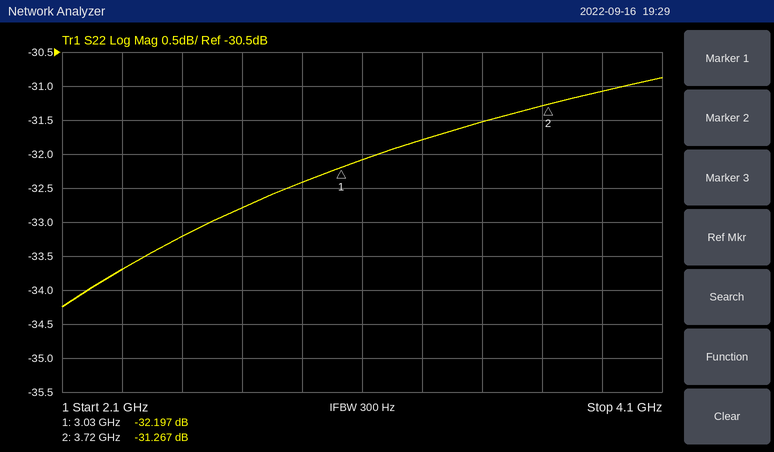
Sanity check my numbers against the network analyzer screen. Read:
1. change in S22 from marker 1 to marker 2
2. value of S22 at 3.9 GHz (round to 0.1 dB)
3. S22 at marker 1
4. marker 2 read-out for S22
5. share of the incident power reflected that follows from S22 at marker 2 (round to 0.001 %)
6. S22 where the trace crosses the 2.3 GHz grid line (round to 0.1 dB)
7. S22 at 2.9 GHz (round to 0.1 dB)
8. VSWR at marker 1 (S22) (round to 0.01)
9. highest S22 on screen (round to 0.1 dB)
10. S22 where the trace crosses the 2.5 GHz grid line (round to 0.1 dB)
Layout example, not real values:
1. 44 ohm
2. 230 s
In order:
1. 0.930 dB
2. -31.1 dB
3. -32.197 dB
4. -31.267 dB
5. 0.075 %
6. -33.7 dB
7. -32.4 dB
8. 1.05
9. -30.9 dB
10. -33.2 dB
